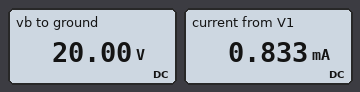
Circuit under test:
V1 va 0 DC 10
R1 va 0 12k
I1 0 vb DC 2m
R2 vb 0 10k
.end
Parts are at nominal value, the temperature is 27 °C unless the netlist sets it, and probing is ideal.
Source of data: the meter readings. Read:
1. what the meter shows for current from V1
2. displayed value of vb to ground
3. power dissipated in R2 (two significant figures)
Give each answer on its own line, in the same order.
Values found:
0.833 mA
20.00 V
40 mW
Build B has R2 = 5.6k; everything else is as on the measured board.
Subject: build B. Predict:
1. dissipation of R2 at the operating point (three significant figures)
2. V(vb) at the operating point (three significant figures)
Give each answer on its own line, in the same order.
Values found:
22.4 mW
11.2 V
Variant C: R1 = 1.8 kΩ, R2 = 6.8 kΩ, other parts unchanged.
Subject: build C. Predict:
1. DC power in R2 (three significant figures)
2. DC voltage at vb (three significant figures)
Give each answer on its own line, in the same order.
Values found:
27.2 mW
13.6 V
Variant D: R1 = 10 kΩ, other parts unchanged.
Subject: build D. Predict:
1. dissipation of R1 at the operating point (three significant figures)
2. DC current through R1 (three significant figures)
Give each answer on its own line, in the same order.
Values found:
10.0 mW
1.00 mA
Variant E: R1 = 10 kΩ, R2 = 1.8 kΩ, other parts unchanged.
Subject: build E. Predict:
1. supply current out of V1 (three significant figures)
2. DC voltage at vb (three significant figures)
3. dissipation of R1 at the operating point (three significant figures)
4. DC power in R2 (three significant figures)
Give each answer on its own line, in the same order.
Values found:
1.00 mA
3.60 V
10.0 mW
7.20 mW
